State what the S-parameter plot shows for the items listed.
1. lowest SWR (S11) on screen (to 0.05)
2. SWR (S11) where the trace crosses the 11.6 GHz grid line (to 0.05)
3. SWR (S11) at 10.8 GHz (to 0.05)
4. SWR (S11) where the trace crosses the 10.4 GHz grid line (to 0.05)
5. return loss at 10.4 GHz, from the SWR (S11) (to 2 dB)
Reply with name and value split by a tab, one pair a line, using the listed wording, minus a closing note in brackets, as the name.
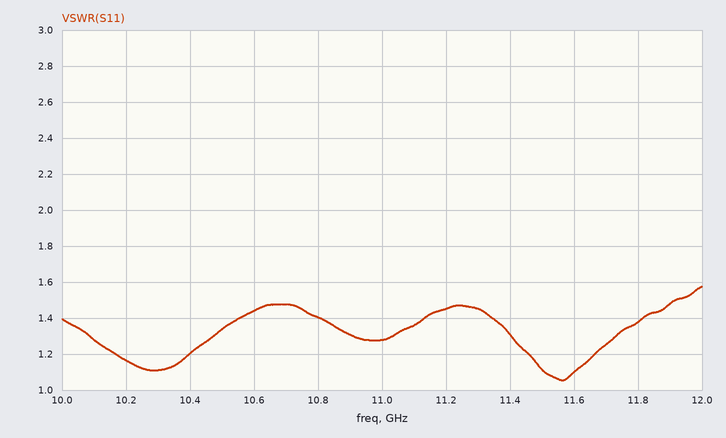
lowest SWR (S11) on screen	1.05
SWR (S11) where the trace crosses the 11.6 GHz grid line	1.10
SWR (S11) at 10.8 GHz	1.40
SWR (S11) where the trace crosses the 10.4 GHz grid line	1.20
return loss at 10.4 GHz, from the SWR (S11)	20 dB
